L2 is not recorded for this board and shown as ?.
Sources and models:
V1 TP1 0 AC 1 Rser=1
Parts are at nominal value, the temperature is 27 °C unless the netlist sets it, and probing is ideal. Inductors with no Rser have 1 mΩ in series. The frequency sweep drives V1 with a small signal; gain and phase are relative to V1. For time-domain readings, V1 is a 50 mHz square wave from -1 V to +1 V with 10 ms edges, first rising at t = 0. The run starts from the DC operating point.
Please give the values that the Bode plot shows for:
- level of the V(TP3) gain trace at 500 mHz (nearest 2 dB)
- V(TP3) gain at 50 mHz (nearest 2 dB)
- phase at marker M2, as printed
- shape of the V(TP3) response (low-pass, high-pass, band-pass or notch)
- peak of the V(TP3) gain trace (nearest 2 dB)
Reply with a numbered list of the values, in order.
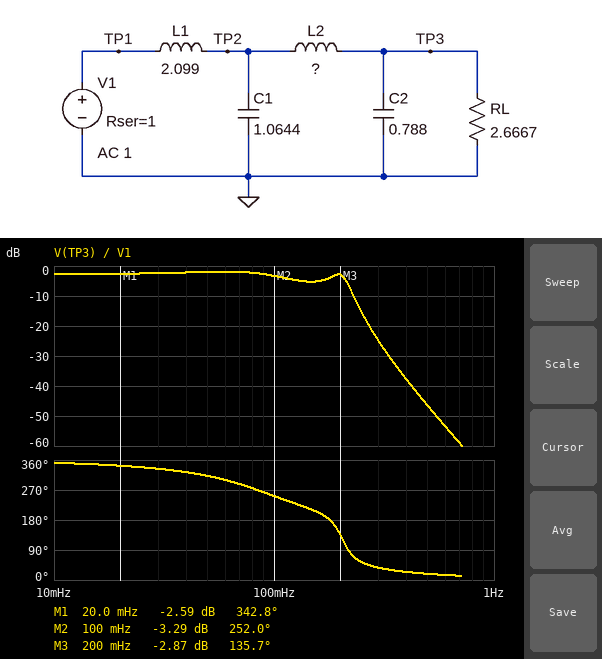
1. -46 dB
2. -2 dB
3. 252.0 deg
4. low-pass
5. -2 dB
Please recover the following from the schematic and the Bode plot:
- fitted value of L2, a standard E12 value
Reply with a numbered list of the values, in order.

1. 1.5 H
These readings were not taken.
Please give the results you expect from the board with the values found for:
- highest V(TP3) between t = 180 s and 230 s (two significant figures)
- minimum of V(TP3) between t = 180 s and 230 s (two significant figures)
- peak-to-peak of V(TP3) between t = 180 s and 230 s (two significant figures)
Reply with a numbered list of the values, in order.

1. 920 mV
2. -920 mV
3. 1.8 V
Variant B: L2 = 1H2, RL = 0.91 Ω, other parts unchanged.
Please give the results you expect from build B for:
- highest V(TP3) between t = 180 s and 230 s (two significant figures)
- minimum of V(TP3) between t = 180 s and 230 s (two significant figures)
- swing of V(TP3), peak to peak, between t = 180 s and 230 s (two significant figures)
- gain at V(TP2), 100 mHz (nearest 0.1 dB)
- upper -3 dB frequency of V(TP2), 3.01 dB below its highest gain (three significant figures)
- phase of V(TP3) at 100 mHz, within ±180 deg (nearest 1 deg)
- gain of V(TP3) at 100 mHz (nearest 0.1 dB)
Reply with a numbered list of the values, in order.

1. 510 mV
2. -510 mV
3. 1.0 V
4. -7.5 dB
5. 234 mHz
6. -91 deg
7. -7.8 dB
